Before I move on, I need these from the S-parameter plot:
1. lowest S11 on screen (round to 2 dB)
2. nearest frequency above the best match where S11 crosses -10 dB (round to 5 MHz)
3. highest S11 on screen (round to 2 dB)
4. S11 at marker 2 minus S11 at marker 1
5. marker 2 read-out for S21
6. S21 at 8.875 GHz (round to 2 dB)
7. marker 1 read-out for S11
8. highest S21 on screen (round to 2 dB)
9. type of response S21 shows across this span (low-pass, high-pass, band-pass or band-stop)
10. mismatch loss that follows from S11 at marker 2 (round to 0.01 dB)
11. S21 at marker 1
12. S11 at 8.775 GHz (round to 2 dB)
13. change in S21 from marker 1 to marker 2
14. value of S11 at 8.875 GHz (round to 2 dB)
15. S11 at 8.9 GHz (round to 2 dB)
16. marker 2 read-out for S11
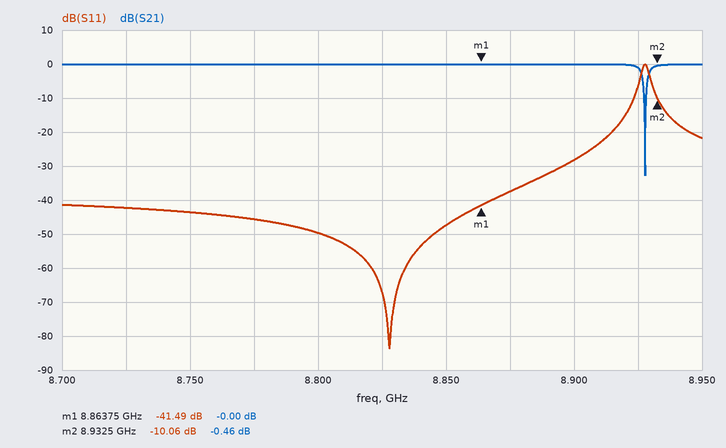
-84 dB
8.925 GHz
0 dB
31.43 dB
-0.46 dB
0 dB
-41.49 dB
0 dB
band-stop
0.45 dB
-0.00 dB
-46 dB
-0.46 dB
-38 dB
-28 dB
-10.06 dB
